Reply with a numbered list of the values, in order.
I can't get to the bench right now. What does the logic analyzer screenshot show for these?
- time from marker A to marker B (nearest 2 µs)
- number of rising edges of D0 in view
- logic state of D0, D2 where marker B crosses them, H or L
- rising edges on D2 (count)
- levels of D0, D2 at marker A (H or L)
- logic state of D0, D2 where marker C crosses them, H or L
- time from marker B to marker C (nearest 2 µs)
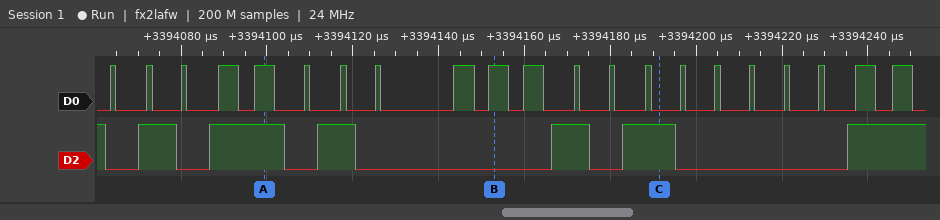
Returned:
1. 54 µs
2. 21
3. D0=H, D2=L
4. 6
5. D0=H, D2=H
6. D0=L, D2=H
7. 38 µs
